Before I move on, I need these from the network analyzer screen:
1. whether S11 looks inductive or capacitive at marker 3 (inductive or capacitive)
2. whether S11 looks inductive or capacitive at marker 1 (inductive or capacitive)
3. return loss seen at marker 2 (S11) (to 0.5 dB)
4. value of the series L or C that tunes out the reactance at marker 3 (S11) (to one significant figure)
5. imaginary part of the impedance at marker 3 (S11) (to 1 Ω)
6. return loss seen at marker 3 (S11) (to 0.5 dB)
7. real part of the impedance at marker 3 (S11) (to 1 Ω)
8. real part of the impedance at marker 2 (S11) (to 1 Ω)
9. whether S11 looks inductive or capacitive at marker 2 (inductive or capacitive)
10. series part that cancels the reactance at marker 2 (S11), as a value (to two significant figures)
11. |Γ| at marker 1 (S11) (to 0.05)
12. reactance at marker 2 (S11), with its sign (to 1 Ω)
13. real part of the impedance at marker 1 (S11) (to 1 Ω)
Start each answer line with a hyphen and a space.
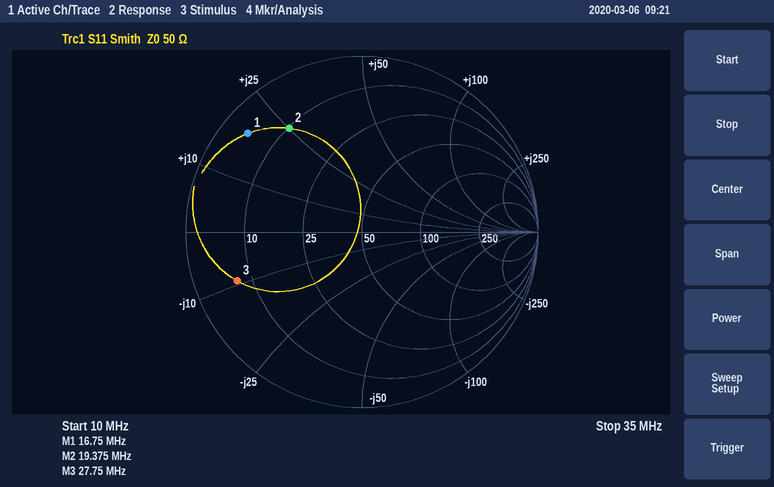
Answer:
- capacitive
- inductive
- 3.0 dB
- 50 nH
- -9 Ω
- 2.5 dB
- 7 Ω
- 10 Ω
- inductive
- 330 pF
- 0.85
- +25 Ω
- 4 Ω
